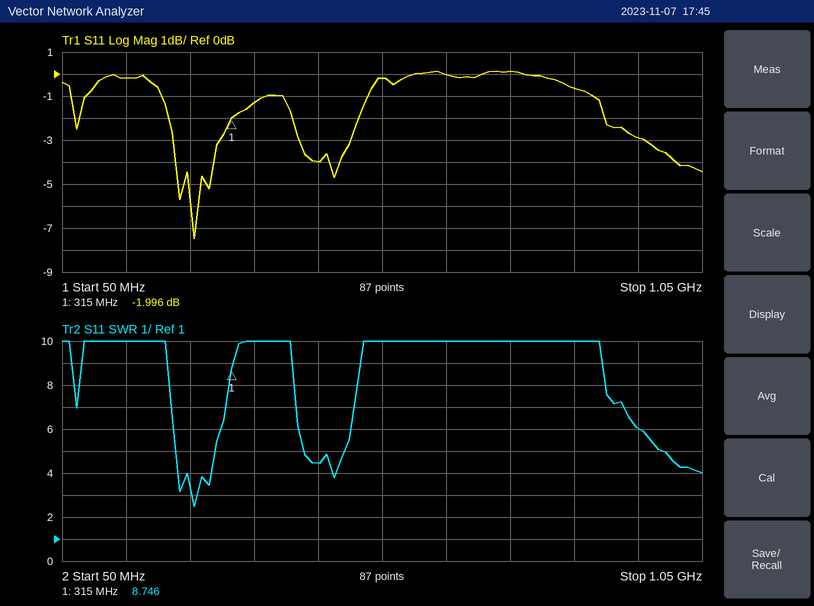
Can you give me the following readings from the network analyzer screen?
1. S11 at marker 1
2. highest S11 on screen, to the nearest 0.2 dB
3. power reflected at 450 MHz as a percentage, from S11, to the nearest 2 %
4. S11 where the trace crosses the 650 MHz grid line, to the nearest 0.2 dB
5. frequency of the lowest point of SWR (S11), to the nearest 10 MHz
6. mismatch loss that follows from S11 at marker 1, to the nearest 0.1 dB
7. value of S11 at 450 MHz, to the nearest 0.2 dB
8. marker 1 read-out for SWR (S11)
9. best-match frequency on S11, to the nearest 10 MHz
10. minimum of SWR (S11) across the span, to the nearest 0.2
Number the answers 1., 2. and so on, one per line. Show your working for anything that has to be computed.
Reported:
1. -1.996 dB
2. 0.2 dB
3. 10^(-4/10) ≈ 40 %
4. 0.0 dB
5. 260 MHz
6. −10 log10(1 − 10^(-1.996/10)) ≈ 4.3 dB
7. -4.0 dB
8. 8.746
9. 260 MHz
10. 2.4
